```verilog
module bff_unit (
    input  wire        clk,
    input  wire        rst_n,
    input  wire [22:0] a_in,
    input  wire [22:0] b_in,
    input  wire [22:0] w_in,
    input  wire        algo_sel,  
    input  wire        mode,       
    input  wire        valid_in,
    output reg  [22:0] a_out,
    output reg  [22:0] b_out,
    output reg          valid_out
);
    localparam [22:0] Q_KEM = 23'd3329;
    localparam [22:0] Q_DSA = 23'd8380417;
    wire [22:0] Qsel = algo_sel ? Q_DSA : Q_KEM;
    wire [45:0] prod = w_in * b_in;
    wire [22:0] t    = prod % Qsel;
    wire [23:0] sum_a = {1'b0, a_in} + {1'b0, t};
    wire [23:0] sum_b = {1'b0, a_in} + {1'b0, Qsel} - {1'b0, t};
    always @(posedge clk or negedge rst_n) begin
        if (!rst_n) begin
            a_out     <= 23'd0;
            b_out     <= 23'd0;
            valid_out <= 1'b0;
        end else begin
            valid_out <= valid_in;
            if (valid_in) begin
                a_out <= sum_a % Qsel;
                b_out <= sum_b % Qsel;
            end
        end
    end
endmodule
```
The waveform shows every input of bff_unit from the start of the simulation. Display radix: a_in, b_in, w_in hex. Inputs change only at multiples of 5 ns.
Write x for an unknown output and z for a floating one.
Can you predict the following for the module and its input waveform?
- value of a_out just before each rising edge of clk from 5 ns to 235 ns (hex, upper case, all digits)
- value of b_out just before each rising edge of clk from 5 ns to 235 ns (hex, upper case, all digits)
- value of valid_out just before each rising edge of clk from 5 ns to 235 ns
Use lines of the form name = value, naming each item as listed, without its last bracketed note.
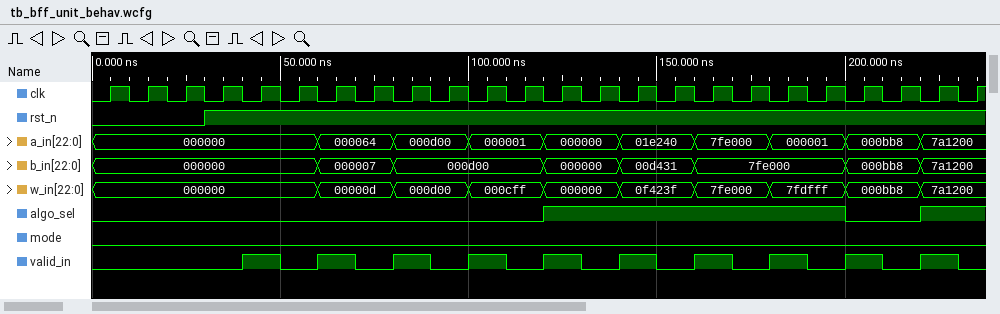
value of a_out just before each rising edge of clk from 5 ns to 235 ns = 000000, 000000, 000000, 000000, 000000, 000000, 000000, 0000BF, 0000BF, 000000, 000000, 000003, 000003, 000000, 000000, 73C2FE, 73C2FE, 000000, 000000, 000003, 000003, 000568, 000568, 380A8C
value of b_out just before each rising edge of clk from 5 ns to 235 ns = 000000, 000000, 000000, 000000, 000000, 000000, 000000, 000009, 000009, 000CFF, 000CFF, 000D00, 000D00, 000000, 000000, 0FE183, 0FE183, 7FDFFF, 7FDFFF, 7FE000, 7FE000, 000507, 000507, 3C3973
value of valid_out just before each rising edge of clk from 5 ns to 235 ns = 0 0 0 0 0 1 0 1 0 1 0 1 0 1 0 1 0 1 0 1 0 1 0 1
